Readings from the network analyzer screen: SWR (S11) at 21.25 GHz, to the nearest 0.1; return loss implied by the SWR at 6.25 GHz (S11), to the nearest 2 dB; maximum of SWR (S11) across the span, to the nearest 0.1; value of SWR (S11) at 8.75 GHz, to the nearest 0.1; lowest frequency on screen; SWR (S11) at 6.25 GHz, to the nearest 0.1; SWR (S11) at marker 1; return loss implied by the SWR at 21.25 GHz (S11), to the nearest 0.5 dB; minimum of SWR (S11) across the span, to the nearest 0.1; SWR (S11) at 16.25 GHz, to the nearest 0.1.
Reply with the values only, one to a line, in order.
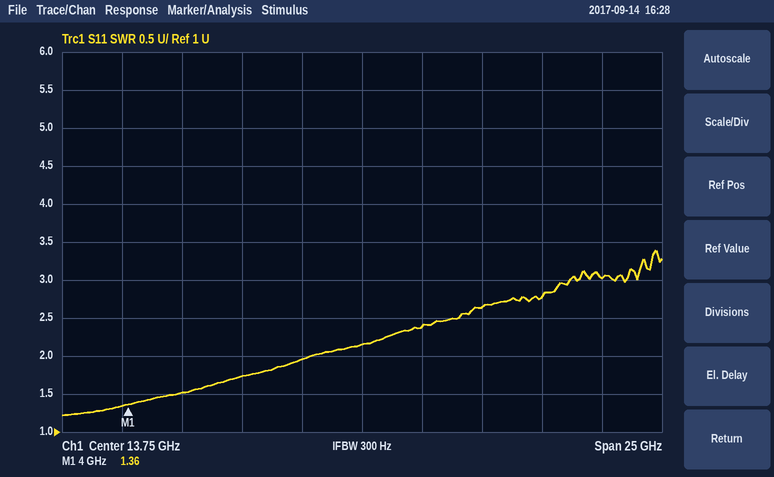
2.8
14 dB
3.4
1.7
1.25 GHz
1.5
1.36
6.5 dB
1.2
2.4
